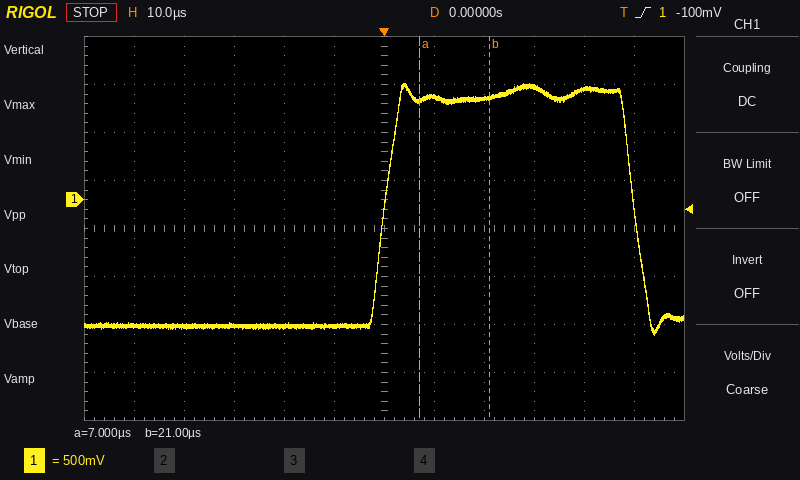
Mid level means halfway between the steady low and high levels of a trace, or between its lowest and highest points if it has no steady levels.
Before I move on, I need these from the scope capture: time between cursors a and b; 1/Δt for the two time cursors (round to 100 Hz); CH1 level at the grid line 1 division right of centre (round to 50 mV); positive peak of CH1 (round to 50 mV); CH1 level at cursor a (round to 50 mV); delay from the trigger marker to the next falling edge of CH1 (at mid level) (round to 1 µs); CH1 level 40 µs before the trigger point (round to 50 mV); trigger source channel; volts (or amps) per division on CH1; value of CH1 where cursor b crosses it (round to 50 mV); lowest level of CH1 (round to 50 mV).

14 µs
71.4 kHz
1.05 V
1.20 V
1.05 V
50 µs
-1.30 V
CH1
500 mV
1.05 V
-1.40 V
